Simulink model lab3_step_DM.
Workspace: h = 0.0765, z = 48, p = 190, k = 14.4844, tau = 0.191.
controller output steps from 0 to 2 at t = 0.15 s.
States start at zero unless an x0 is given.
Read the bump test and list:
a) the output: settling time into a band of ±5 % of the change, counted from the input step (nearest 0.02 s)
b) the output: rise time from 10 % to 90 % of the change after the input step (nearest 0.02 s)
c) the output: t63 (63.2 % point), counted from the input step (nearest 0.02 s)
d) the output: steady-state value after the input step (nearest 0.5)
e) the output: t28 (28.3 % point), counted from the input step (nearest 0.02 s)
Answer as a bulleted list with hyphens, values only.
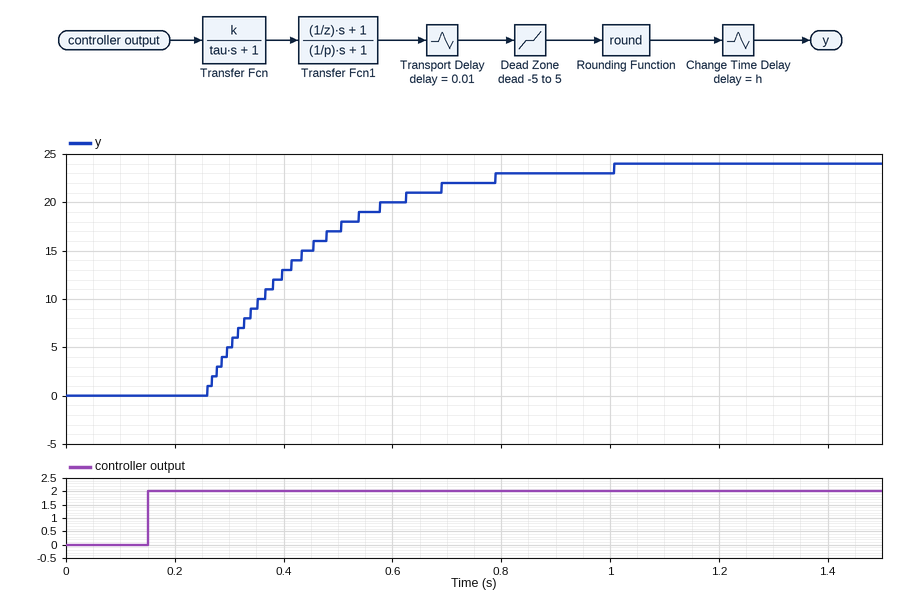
- 0.64 s
- 0.42 s
- 0.30 s
- 24.0
- 0.16 s
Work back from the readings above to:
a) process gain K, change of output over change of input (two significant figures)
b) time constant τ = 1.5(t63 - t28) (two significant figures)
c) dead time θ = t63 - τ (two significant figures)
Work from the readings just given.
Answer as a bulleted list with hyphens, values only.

- 12
- 0.21 s
- 0.090 s
